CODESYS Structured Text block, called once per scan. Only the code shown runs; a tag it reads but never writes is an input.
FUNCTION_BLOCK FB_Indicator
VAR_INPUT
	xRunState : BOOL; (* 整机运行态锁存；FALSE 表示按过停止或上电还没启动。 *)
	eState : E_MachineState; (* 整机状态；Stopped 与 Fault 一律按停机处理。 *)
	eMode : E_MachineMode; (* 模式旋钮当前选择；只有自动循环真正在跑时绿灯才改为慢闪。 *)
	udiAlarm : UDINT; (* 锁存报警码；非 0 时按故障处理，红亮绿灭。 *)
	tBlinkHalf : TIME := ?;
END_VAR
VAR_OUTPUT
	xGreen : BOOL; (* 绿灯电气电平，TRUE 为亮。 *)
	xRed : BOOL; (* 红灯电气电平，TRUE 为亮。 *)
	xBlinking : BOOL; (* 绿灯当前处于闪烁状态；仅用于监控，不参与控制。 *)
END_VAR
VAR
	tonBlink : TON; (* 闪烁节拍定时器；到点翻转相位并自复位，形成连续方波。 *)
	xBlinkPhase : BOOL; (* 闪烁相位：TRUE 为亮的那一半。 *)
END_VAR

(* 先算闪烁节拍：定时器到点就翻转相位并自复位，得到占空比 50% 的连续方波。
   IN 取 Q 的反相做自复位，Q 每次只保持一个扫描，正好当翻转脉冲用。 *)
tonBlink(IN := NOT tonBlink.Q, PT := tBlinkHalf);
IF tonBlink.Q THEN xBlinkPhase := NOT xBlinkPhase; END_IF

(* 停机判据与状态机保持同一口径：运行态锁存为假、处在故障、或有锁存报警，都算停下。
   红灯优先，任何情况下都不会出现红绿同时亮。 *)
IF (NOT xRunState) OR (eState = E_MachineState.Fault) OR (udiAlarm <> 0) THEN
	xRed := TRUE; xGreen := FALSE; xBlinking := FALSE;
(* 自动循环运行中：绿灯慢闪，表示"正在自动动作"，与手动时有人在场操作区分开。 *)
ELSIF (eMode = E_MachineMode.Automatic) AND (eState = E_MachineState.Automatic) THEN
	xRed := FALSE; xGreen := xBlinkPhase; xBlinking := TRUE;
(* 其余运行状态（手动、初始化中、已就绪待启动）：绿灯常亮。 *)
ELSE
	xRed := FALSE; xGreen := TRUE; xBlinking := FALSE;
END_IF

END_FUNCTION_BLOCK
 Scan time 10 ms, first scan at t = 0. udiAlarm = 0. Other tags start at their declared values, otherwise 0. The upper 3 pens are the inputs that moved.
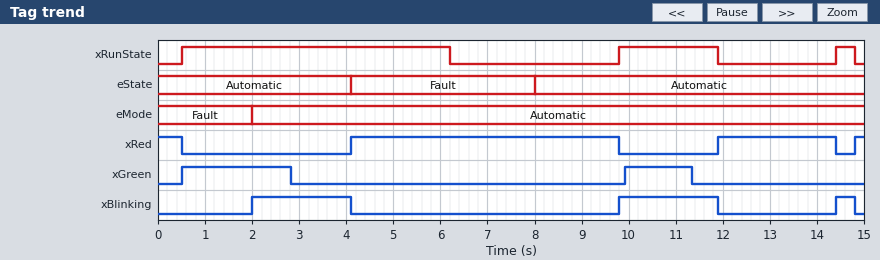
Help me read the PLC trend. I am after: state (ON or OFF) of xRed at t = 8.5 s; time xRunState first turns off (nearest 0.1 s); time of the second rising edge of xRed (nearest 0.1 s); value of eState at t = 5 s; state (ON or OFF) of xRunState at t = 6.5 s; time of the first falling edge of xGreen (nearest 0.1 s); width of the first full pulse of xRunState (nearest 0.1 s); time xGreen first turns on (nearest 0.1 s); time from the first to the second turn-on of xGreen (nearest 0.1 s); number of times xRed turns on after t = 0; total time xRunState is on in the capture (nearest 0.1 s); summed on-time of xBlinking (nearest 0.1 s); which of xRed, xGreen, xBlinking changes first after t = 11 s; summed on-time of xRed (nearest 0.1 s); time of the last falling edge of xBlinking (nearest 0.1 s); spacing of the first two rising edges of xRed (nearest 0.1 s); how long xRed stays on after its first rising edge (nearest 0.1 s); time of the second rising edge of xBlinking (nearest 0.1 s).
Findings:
ON
6.2 s
11.9 s
Fault
OFF
2.8 s
5.7 s
0.5 s
9.4 s
3
8.2 s
4.6 s
xGreen
8.9 s
14.8 s
7.8 s
5.7 s
9.8 s
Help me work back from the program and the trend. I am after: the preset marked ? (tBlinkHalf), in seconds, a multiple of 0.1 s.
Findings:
1.4 s
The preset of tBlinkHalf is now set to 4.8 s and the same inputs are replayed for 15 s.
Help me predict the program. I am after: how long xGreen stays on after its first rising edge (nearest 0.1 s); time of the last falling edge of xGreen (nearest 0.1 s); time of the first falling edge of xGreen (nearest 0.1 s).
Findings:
1.5 s
14.8 s
2.0 s
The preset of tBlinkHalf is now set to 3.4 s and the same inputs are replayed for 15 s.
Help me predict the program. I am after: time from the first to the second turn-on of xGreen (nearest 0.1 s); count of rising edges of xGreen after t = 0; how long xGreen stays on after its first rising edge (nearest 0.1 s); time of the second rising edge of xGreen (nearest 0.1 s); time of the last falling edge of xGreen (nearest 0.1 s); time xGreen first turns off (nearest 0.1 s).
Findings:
2.9 s
3
1.5 s
3.4 s
11.9 s
2.0 s
